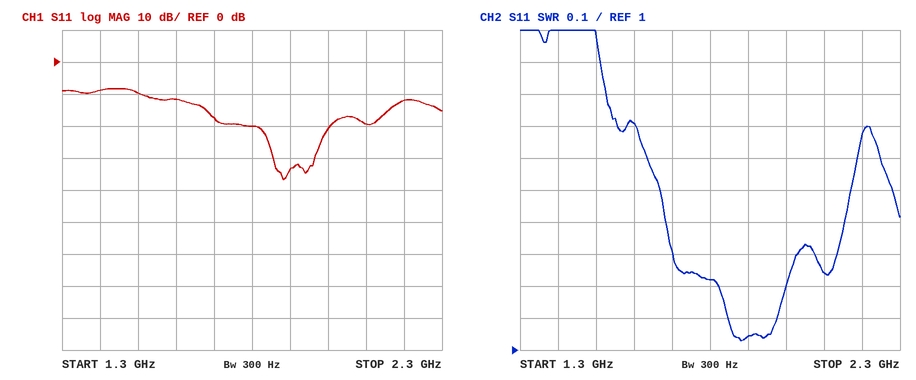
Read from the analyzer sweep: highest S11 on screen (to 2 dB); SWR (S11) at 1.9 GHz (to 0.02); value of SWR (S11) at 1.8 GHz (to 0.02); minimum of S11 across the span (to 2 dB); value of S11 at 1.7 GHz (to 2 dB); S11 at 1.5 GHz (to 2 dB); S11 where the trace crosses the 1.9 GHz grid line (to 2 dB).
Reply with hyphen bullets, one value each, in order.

- -8 dB
- 1.04
- 1.22
- -36 dB
- -18 dB
- -10 dB
- -34 dB
